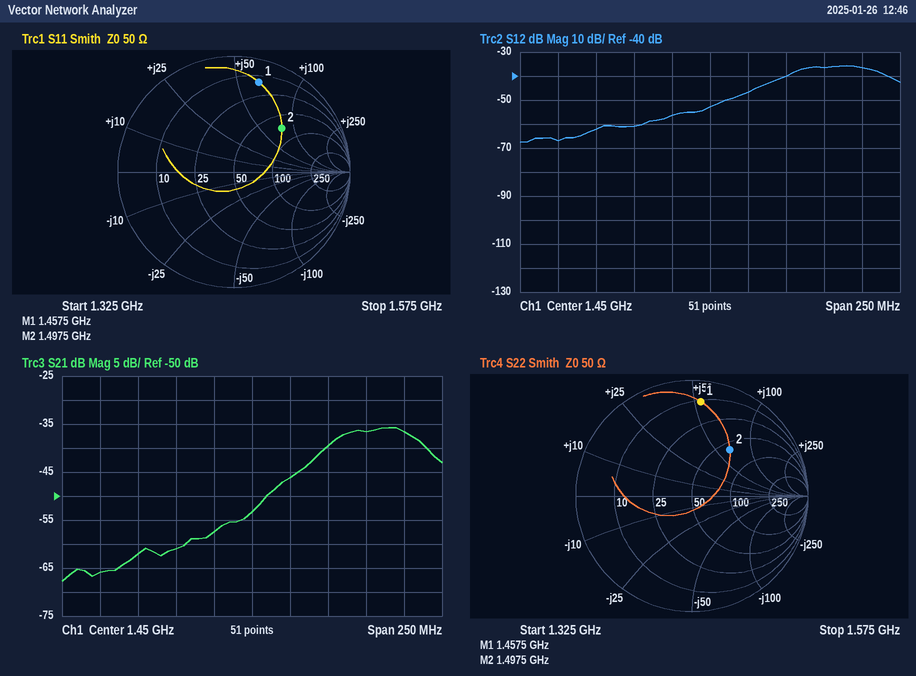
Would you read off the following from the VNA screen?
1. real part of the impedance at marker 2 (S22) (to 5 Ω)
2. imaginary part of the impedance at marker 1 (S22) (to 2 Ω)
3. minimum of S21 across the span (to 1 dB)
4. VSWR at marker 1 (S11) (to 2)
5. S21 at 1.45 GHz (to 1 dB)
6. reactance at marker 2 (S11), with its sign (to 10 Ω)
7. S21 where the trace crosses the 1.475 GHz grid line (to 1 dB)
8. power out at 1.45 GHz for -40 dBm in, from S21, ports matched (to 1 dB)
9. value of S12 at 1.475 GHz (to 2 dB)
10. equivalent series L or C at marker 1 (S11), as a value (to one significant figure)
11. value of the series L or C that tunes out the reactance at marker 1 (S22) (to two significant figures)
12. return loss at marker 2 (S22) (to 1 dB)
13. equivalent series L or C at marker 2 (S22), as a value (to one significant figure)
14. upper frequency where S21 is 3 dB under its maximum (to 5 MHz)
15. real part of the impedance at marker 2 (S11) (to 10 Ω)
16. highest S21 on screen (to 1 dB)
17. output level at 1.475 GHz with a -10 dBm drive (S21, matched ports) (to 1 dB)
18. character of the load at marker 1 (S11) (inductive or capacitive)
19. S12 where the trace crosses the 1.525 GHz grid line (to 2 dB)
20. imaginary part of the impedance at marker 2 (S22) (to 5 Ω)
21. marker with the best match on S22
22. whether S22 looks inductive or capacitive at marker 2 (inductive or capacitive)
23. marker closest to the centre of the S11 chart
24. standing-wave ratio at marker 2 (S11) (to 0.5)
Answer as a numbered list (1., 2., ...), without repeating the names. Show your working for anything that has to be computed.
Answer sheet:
1. 60 Ω
2. +54 Ω
3. -68 dB
4. 10
5. -53 dB
6. +80 Ω
7. -46 dB
8. -40 dBm + (-53 dB) = -93 dBm
9. -46 dB
10. L = 65 Ω/(2π × 1.4575 GHz) ≈ 7 nH
11. C = 1/(2π × 1.4575 GHz × 54 Ω) ≈ 2.0 pF
12. 6 dB
13. L = 65 Ω/(2π × 1.4975 GHz) ≈ 7 nH
14. 1.560 GHz
15. 70 Ω
16. -36 dB
17. -10 dBm + (-46 dB) = -56 dBm
18. inductive
19. -36 dB
20. +65 Ω
21. marker 2
22. inductive
23. marker 2
24. 3.5
